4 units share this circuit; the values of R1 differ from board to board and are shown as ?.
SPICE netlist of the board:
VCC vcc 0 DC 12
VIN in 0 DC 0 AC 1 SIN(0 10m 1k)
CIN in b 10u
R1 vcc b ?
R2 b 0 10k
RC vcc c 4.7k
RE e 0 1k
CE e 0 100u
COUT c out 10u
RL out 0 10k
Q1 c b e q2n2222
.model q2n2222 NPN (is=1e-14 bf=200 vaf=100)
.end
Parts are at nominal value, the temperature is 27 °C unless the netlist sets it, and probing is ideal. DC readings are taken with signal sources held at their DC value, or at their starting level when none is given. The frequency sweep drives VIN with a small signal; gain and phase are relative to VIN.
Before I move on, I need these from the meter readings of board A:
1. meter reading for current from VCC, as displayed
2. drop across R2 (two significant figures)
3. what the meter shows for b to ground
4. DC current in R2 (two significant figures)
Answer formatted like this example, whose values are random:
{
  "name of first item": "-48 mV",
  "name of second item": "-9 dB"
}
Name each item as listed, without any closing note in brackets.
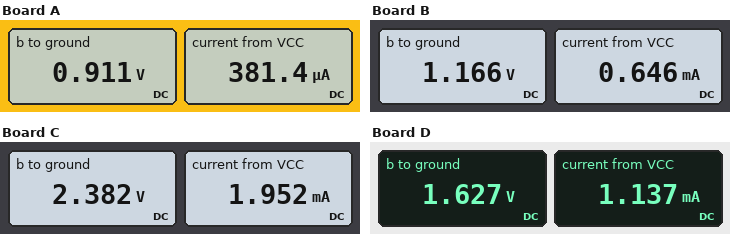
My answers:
{
  "meter reading for current from VCC, as displayed": "381.4 µA",
  "drop across R2": "910 mV",
  "what the meter shows for b to ground": "0.911 V",
  "DC current in R2": "91 µA"
}
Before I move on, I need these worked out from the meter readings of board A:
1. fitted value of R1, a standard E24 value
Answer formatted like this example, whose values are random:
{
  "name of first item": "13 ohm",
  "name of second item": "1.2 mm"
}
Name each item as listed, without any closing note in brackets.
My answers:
{
  "fitted value of R1, a standard E24 value": "120 kΩ"
}
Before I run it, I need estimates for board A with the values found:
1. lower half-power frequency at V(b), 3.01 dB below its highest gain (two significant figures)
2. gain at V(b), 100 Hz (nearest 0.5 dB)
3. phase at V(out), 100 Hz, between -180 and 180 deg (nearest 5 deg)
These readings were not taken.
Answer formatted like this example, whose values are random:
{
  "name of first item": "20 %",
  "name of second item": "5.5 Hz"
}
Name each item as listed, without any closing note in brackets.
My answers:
{
  "lower half-power frequency at V(b), 3.01 dB below its highest gain": "1.9 Hz",
  "gain at V(b), 100 Hz": "0 dB",
  "phase at V(out), 100 Hz, between -180 and 180 deg": "-170 deg"
}
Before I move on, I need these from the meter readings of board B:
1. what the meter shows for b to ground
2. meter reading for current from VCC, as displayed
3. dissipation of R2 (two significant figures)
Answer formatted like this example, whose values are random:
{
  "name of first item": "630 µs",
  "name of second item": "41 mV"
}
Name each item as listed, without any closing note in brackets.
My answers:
{
  "what the meter shows for b to ground": "1.166 V",
  "meter reading for current from VCC, as displayed": "0.646 mA",
  "dissipation of R2": "140 µW"
}
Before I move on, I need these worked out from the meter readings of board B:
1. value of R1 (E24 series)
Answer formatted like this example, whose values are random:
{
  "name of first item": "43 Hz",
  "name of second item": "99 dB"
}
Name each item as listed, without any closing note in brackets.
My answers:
{
  "value of R1": "91 kΩ"
}
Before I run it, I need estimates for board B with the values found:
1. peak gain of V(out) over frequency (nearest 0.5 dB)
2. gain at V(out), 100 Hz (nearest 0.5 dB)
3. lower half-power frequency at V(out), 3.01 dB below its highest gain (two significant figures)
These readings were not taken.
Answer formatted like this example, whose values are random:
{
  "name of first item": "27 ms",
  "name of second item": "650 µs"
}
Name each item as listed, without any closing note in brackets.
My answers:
{
  "peak gain of V(out) over frequency": "36.0 dB",
  "gain at V(out), 100 Hz": "35.5 dB",
  "lower half-power frequency at V(out), 3.01 dB below its highest gain": "35 Hz"
}
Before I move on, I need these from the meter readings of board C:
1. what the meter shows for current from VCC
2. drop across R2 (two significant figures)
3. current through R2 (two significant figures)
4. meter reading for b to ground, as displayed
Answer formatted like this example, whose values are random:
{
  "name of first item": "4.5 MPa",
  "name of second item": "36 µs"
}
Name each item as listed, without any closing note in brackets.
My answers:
{
  "what the meter shows for current from VCC": "1.952 mA",
  "drop across R2": "2.4 V",
  "current through R2": "240 µA",
  "meter reading for b to ground, as displayed": "2.382 V"
}
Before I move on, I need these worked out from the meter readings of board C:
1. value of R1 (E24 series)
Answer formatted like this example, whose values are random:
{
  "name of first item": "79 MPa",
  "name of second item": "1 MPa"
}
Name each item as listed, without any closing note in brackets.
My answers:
{
  "value of R1": "39 kΩ"
}
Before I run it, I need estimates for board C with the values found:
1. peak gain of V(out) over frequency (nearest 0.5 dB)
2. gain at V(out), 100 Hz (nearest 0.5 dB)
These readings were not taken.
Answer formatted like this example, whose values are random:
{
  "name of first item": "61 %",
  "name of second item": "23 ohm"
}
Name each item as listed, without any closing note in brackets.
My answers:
{
  "peak gain of V(out) over frequency": "46.0 dB",
  "gain at V(out), 100 Hz": "42.5 dB"
}
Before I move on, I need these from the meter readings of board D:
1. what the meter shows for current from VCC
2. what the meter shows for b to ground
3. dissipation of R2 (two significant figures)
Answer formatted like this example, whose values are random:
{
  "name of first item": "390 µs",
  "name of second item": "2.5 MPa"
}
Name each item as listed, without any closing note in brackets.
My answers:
{
  "what the meter shows for current from VCC": "1.137 mA",
  "what the meter shows for b to ground": "1.627 V",
  "dissipation of R2": "260 µW"
}
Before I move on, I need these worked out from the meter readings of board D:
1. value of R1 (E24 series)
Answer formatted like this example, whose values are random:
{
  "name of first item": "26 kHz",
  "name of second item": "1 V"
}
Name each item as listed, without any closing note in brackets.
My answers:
{
  "value of R1": "62 kΩ"
}
